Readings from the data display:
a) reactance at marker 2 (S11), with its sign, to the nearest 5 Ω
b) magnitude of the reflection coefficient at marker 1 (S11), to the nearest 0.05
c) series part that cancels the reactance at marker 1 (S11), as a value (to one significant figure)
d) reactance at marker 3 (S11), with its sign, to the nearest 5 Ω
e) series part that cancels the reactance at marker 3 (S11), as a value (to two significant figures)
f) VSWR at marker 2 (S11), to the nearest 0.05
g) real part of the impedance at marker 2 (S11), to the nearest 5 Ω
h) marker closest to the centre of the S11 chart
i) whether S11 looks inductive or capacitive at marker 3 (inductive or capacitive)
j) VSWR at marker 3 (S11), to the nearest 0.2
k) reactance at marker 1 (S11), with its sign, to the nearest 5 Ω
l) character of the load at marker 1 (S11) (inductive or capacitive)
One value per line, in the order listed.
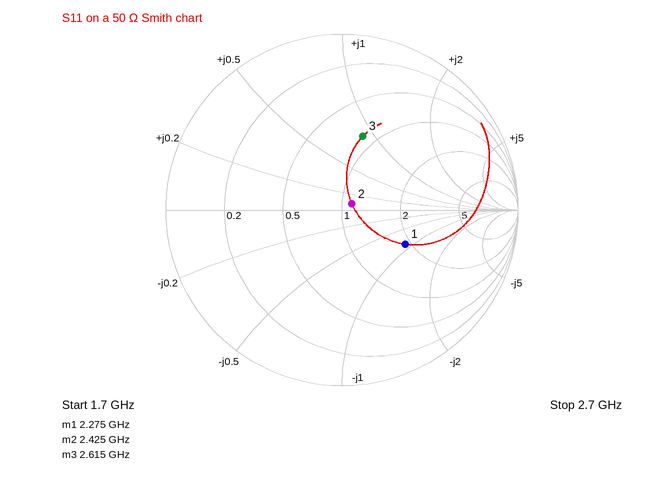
+5 Ω
0.40
3 nH
+45 Ω
1.4 pF
1.15
55 Ω
marker 2
inductive
2.6
-45 Ω
capacitive
